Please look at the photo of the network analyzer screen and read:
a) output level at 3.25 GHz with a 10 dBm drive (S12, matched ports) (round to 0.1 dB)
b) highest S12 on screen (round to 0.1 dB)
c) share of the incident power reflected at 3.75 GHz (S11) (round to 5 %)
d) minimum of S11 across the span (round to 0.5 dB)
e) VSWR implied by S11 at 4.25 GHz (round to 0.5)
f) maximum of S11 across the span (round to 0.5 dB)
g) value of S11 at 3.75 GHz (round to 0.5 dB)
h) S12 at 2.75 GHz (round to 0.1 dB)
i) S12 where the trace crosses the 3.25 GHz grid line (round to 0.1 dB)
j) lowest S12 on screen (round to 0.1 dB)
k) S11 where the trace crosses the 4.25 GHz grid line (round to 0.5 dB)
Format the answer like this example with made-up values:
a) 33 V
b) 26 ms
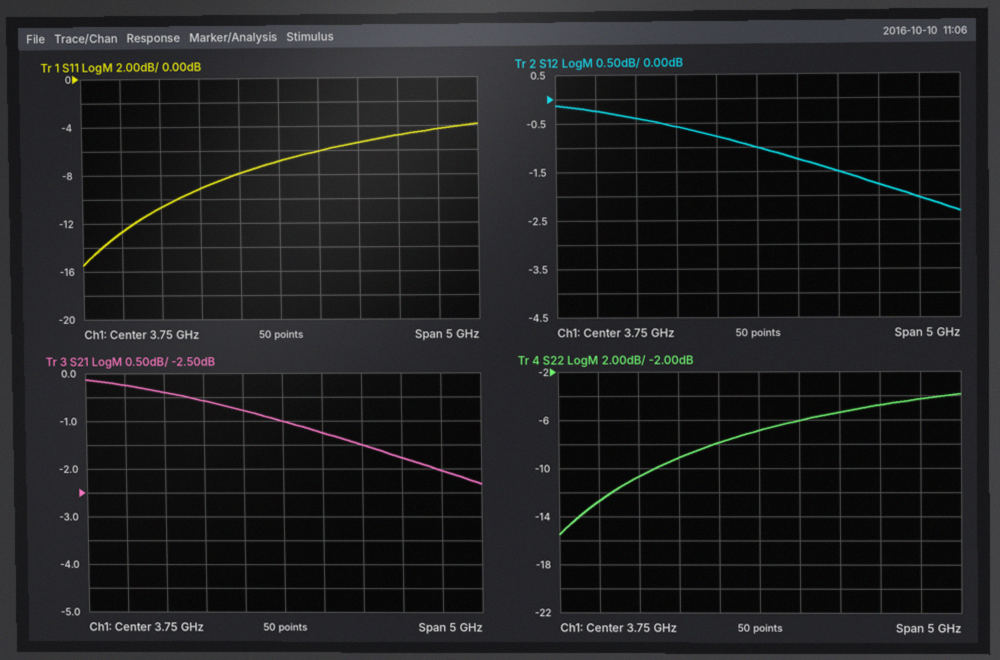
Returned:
a) 9.2 dBm
b) -0.1 dB
c) 20 %
d) -15.5 dB
e) 3.0
f) -4.0 dB
g) -7.0 dB
h) -0.6 dB
i) -0.8 dB
j) -2.3 dB
k) -6.0 dB
